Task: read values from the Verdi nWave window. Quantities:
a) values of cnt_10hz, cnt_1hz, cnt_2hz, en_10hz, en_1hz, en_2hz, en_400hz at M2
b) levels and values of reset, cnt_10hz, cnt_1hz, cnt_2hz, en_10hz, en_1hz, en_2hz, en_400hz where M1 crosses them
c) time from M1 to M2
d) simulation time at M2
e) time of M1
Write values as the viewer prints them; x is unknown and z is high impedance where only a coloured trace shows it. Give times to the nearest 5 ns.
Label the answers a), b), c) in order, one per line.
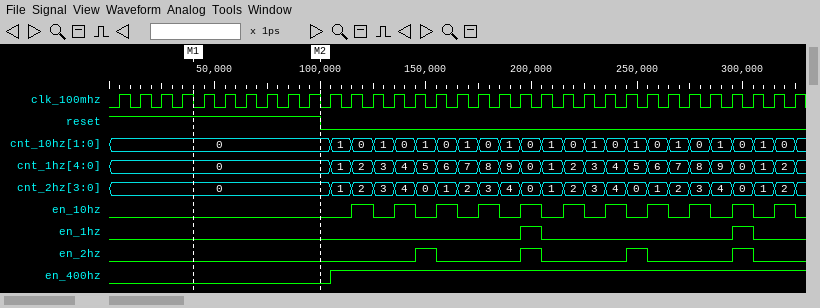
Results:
a) cnt_10hz=0, cnt_1hz=0, cnt_2hz=0, en_10hz=0, en_1hz=0, en_2hz=0, en_400hz=0
b) reset=1, cnt_10hz=0, cnt_1hz=0, cnt_2hz=0, en_10hz=0, en_1hz=0, en_2hz=0, en_400hz=0
c) 60 ns
d) 100 ns
e) 40 ns
